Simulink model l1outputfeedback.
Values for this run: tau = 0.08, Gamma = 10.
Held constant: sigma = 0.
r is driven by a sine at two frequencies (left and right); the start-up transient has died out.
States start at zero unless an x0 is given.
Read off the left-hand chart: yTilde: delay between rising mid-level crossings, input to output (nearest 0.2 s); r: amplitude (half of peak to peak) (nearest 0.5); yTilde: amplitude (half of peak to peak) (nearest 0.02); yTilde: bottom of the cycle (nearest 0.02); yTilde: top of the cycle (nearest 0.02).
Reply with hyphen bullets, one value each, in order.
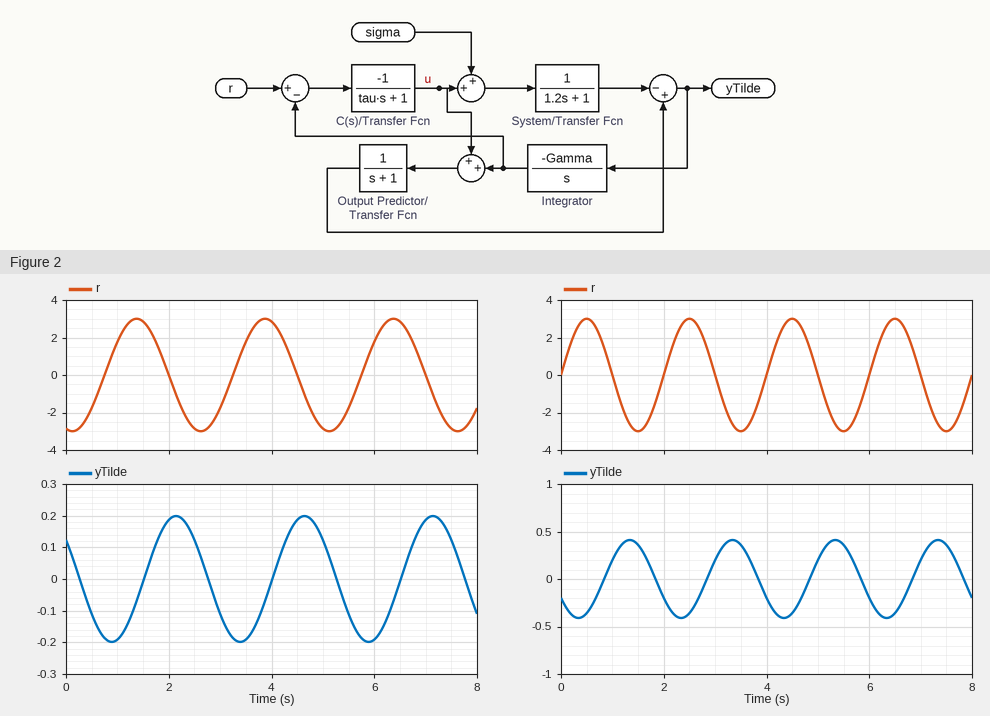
- 0.8 s
- 3.0
- 0.20
- -0.20
- 0.20
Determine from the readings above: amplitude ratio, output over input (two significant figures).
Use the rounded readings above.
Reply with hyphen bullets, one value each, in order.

- 0.067
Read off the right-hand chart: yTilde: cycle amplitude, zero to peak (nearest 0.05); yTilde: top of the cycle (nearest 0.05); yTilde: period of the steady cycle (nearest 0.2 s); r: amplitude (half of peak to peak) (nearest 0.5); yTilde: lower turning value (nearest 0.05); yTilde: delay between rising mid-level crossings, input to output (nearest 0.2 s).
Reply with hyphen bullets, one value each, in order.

- 0.40
- 0.40
- 2.0 s
- 3.0
- -0.40
- 0.8 s
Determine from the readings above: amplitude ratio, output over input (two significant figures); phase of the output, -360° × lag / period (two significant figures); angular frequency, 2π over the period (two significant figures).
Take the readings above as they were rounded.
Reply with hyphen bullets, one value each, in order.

- 0.13
- -140°
- 3.1 rad/s
